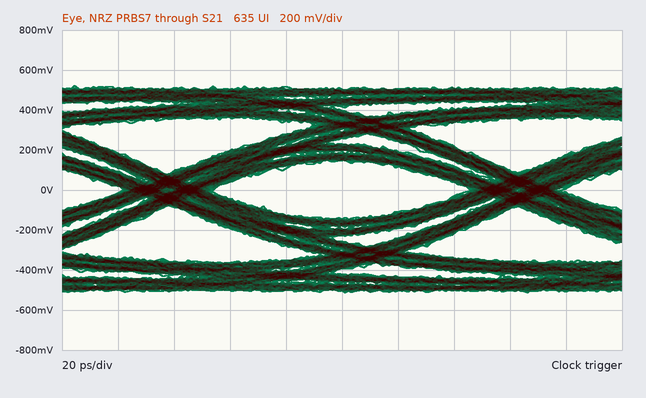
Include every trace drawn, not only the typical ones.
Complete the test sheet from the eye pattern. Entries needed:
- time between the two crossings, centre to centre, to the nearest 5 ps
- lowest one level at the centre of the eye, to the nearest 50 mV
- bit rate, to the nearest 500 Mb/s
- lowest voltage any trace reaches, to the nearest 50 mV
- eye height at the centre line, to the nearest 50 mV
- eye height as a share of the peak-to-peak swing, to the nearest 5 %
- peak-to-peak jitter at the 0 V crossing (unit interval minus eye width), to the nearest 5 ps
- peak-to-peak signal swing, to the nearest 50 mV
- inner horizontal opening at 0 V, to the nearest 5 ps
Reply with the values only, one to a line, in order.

125 ps
150 mV
8.0 Gb/s
-500 mV
300 mV
30 %
35 ps
1.05 V
90 ps
